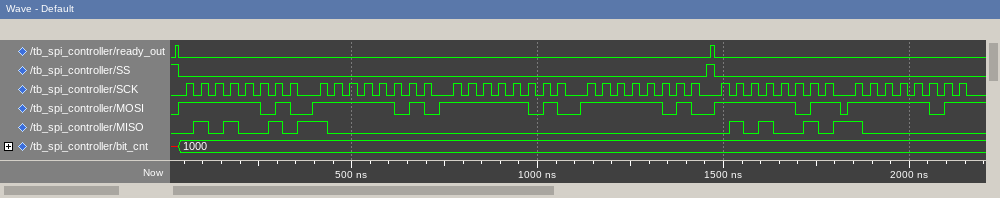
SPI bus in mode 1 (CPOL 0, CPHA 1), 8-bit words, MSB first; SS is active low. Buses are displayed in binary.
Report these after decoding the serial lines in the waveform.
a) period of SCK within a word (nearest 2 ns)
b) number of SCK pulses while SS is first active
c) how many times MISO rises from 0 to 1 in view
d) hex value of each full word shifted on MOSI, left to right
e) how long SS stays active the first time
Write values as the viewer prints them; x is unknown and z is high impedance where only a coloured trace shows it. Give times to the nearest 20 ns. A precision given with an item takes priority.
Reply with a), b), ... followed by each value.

a) 40 ns
b) 32
c) 8
d) FA, FA, FA, FA, FB, FB
e) 1420 ns
